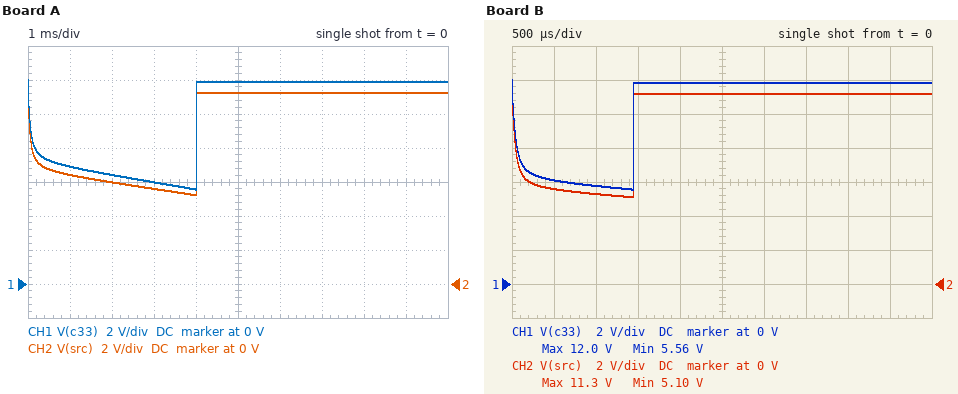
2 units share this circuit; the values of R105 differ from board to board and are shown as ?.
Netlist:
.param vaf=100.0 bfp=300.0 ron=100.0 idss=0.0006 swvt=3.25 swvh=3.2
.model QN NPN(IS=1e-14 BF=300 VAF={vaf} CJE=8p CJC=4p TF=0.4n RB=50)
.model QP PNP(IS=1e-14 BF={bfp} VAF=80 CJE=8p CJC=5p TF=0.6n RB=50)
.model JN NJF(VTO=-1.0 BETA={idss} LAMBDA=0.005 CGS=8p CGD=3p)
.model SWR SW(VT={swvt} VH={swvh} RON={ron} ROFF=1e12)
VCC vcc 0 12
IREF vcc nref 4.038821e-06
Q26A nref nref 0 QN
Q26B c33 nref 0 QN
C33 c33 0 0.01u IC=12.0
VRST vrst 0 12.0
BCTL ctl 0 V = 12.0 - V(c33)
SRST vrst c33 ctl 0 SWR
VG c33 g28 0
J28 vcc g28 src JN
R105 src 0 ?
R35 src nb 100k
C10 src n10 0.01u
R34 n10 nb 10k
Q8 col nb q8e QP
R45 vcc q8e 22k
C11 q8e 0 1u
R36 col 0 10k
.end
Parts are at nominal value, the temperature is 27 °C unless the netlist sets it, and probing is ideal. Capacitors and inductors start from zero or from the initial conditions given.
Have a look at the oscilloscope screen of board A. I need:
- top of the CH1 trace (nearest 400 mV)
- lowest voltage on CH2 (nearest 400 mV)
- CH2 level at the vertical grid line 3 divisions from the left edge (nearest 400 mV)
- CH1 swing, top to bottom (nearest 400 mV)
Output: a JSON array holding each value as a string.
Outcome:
["12.0 V", "5.2 V", "5.6 V", "6.4 V"]
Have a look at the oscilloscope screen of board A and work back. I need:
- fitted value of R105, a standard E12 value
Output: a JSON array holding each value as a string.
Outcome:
["4.7 kΩ"]
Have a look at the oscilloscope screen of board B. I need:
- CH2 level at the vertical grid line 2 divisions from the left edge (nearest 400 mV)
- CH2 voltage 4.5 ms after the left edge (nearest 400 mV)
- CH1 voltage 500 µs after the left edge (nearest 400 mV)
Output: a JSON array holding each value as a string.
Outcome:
["5.2 V", "11.2 V", "6.0 V"]
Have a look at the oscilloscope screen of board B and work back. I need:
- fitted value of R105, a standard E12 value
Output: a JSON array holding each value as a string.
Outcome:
["3.9 kΩ"]
